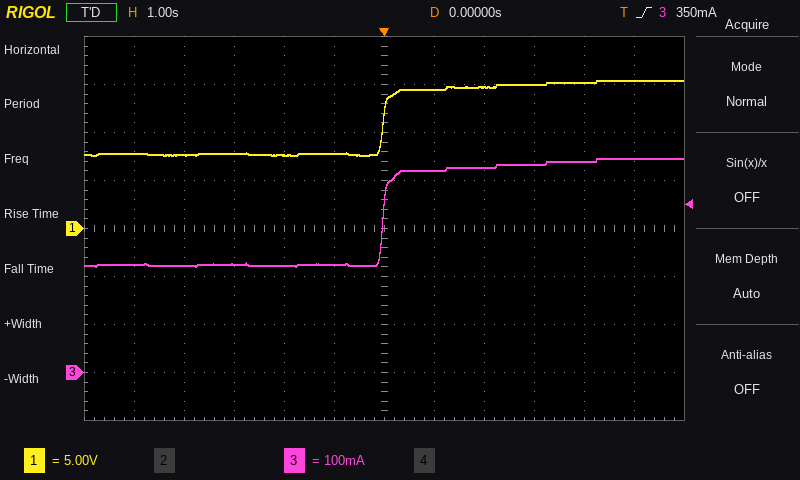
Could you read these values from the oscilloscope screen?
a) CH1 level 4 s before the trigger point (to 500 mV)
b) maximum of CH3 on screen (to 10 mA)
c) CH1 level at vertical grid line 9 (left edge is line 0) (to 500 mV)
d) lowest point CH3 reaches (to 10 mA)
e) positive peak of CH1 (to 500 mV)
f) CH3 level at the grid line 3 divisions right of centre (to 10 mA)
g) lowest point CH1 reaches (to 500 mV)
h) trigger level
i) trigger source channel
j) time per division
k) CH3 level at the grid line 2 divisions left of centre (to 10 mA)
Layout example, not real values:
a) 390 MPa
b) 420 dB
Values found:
a) 7.5 V
b) 450 mA
c) 15.0 V
d) 220 mA
e) 15.5 V
f) 430 mA
g) 7.5 V
h) 350 mA
i) CH3
j) 1 s
k) 220 mA
